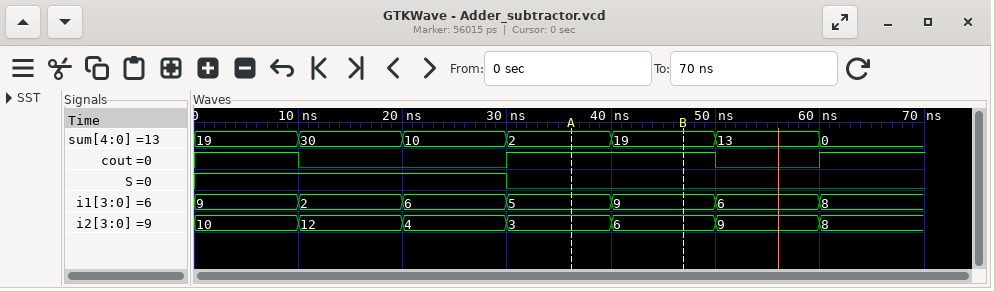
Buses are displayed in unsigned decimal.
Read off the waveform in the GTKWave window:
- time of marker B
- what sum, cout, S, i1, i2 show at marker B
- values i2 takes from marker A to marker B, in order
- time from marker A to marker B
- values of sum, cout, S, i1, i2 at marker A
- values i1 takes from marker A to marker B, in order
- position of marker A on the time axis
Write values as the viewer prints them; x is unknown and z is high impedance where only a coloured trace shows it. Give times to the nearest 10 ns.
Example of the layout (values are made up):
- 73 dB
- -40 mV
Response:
- 50 ns
- sum=19, cout=1, S=0, i1=9, i2=6
- 3, 6
- 10 ns
- sum=2, cout=1, S=0, i1=5, i2=3
- 5, 9
- 40 ns
